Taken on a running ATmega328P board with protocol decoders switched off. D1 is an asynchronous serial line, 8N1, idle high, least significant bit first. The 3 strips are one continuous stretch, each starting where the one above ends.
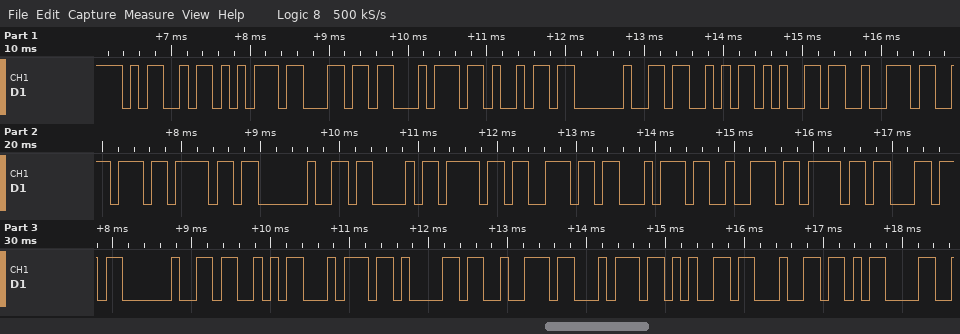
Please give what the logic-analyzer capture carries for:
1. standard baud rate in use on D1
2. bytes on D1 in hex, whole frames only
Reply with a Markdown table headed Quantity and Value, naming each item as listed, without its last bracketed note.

| Quantity | Value |
|---|---|
| standard baud rate in use on D1 | 9600 baud |
| bytes on D1 in hex, whole frames only | 4D 75 6C 74 69 20 53 65 72 76 6F 20 43 6F 6E 74 72 6F 6C 20 53 74 61 72 74 65 64 0D |
